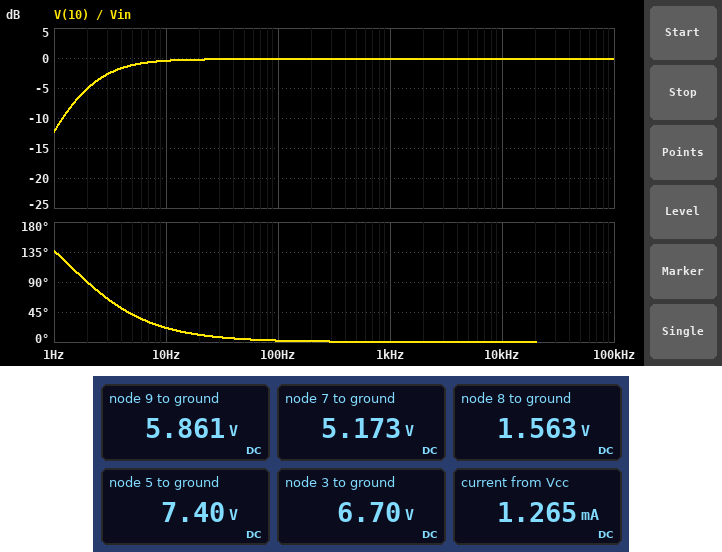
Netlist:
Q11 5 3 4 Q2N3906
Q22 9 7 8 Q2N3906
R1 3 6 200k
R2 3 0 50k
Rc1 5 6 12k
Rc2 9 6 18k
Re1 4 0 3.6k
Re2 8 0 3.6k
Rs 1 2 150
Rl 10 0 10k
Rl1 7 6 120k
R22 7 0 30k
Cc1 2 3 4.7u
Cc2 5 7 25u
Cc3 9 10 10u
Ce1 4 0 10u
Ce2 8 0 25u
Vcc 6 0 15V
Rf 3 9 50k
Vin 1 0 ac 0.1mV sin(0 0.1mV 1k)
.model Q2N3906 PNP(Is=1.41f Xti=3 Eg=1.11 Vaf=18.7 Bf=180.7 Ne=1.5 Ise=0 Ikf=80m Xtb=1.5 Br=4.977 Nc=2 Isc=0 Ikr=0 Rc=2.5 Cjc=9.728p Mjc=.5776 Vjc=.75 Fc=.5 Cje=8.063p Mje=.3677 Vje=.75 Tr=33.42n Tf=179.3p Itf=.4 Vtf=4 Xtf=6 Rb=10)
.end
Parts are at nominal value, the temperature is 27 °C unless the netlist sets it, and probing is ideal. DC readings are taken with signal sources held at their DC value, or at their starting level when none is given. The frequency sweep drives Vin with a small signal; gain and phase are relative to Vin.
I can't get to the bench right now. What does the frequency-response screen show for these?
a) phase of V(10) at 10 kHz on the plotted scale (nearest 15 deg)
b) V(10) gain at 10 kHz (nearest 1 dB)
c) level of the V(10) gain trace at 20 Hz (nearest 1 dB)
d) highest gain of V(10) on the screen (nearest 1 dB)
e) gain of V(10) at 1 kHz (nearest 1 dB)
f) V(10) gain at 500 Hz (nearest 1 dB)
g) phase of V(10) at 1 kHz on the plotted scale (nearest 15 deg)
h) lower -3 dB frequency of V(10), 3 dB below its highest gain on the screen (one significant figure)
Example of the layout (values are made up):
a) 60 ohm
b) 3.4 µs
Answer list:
a) 0 deg
b) 0 dB
c) 0 dB
d) 0 dB
e) 0 dB
f) 0 dB
g) 0 deg
h) 3 Hz
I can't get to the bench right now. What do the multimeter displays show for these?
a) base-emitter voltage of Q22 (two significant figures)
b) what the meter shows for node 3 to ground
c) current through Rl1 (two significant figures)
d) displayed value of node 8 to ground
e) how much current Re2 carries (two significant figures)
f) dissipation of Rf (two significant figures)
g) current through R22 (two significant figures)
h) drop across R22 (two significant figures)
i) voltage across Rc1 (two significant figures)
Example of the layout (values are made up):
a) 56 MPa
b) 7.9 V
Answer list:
a) 3.6 V
b) 6.70 V
c) 82 µA
d) 1.563 V
e) 430 µA
f) 14 µW
g) 170 µA
h) 5.2 V
i) 7.6 V
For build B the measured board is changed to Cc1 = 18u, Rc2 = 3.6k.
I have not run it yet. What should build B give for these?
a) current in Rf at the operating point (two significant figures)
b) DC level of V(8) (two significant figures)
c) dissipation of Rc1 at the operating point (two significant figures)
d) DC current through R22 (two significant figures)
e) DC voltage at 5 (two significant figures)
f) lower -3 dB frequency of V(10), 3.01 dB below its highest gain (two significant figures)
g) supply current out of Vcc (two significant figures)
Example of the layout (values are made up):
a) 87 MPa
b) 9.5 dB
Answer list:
a) 34 µA
b) 4.3 V
c) 3.3 mW
d) 300 µA
e) 8.7 V
f) 2.0 Hz
g) 2.1 mA
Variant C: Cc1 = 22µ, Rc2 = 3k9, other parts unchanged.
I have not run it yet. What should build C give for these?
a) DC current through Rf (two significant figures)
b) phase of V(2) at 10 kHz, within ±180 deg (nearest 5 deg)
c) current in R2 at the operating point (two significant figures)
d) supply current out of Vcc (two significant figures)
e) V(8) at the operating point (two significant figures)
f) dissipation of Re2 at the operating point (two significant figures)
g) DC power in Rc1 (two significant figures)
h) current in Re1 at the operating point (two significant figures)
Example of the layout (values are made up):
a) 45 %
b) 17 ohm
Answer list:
a) 31 µA
b) 0 deg
c) 160 µA
d) 2.0 mA
e) 4.1 V
f) 4.7 mW
g) 3.4 mW
h) 440 µA
